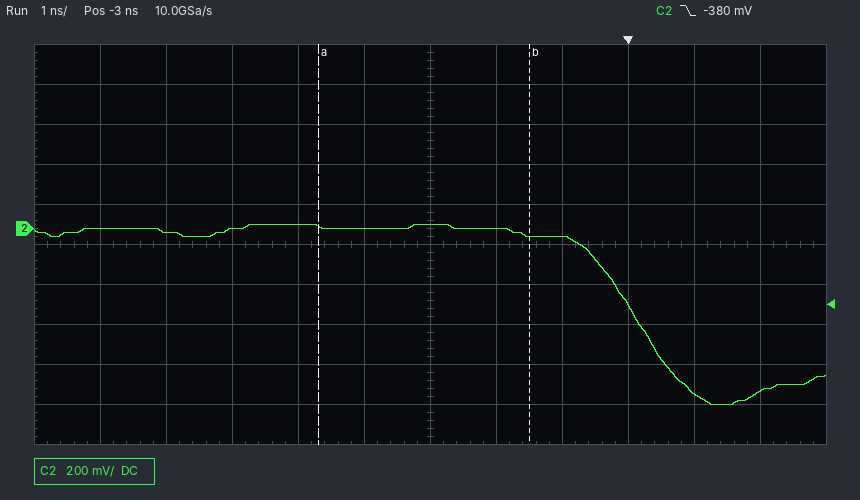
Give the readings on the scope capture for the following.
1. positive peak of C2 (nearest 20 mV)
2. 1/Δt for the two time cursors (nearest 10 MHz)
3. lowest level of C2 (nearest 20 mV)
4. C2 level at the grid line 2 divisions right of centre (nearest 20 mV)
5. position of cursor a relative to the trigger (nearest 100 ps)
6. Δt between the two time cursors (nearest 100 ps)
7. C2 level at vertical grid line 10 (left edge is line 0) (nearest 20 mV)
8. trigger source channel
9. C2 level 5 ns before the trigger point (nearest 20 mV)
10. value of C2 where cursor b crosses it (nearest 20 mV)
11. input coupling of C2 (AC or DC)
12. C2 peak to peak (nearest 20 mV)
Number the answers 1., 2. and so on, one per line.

1. 20 mV
2. 310 MHz
3. -880 mV
4. -40 mV
5. -4.7 ns
6. 3.2 ns
7. -820 mV
8. C2
9. 20 mV
10. -40 mV
11. DC
12. 900 mV
